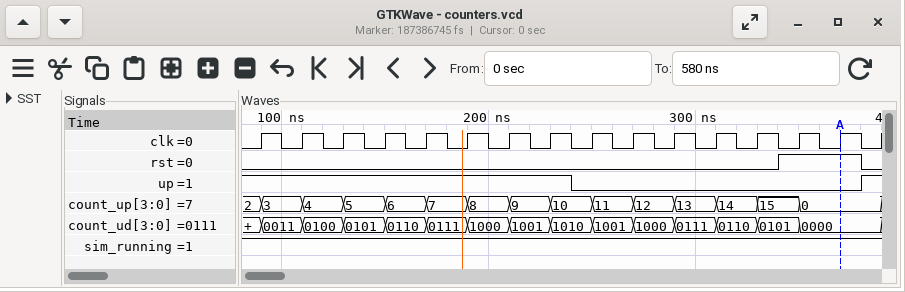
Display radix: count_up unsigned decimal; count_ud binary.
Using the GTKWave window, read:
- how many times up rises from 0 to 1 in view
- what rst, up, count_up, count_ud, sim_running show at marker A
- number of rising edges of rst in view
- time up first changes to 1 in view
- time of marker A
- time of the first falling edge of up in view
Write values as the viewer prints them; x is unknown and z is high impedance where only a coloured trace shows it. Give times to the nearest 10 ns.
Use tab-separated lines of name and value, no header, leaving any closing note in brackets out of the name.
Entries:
how many times up rises from 0 to 1 in view	1
what rst, up, count_up, count_ud, sim_running show at marker A	rst=1, up=0, count_up=0, count_ud=0000, sim_running=1
number of rising edges of rst in view	1
time up first changes to 1 in view	380 ns
time of marker A	370 ns
time of the first falling edge of up in view	240 ns
